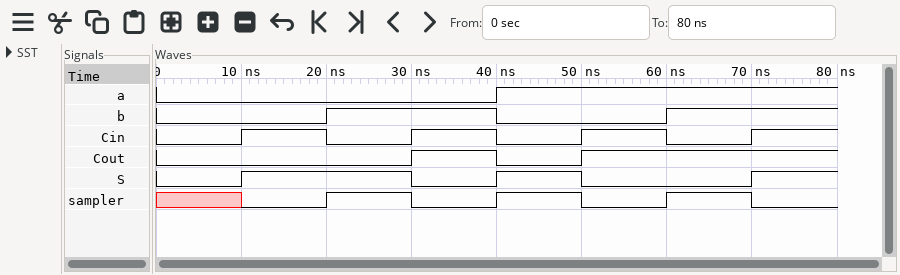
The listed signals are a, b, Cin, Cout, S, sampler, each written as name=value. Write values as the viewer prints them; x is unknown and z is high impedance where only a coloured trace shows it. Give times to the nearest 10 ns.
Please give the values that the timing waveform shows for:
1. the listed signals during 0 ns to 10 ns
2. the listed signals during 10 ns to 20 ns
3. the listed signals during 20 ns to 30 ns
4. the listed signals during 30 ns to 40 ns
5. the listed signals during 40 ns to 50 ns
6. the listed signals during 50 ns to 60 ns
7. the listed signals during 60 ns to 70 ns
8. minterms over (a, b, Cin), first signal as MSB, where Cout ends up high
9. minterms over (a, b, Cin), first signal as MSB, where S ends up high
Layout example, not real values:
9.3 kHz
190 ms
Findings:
a=0, b=0, Cin=0, Cout=0, S=0, sampler=x
a=0, b=0, Cin=1, Cout=0, S=1, sampler=0
a=0, b=1, Cin=0, Cout=0, S=1, sampler=1
a=0, b=1, Cin=1, Cout=1, S=0, sampler=0
a=1, b=0, Cin=0, Cout=0, S=1, sampler=1
a=1, b=0, Cin=1, Cout=1, S=0, sampler=0
a=1, b=1, Cin=0, Cout=1, S=0, sampler=1
3, 5, 6, 7
1, 2, 4, 7
